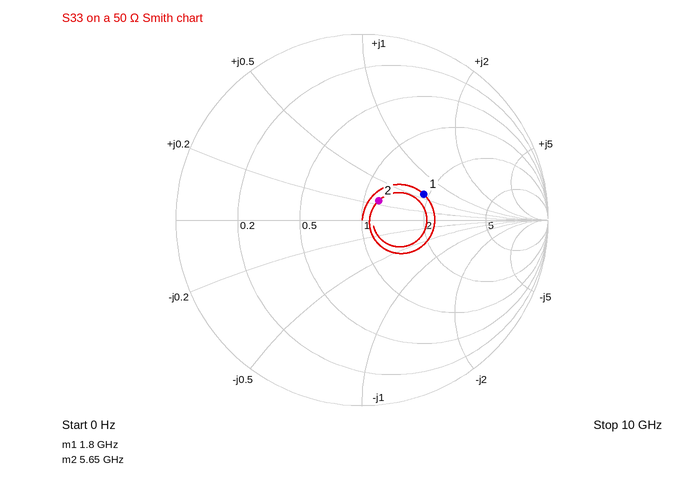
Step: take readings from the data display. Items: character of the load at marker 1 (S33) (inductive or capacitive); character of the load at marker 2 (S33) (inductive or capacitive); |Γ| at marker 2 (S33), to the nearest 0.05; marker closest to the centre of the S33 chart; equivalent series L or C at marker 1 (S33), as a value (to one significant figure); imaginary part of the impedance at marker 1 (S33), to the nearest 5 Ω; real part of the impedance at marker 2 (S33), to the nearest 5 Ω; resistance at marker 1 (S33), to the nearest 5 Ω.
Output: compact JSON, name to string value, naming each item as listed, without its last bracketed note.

{"character of the load at marker 1 (S33)": "inductive", "character of the load at marker 2 (S33)": "inductive", "|Γ| at marker 2 (S33), to the nearest 0.05": "0.15", "marker closest to the centre of the S33 chart": "marker 2", "equivalent series L or C at marker 1 (S33), as a value": "3 nH", "imaginary part of the impedance at marker 1 (S33), to the nearest 5 Ω": "+30 Ω", "real part of the impedance at marker 2 (S33), to the nearest 5 Ω": "60 Ω", "resistance at marker 1 (S33), to the nearest 5 Ω": "95 Ω"}
